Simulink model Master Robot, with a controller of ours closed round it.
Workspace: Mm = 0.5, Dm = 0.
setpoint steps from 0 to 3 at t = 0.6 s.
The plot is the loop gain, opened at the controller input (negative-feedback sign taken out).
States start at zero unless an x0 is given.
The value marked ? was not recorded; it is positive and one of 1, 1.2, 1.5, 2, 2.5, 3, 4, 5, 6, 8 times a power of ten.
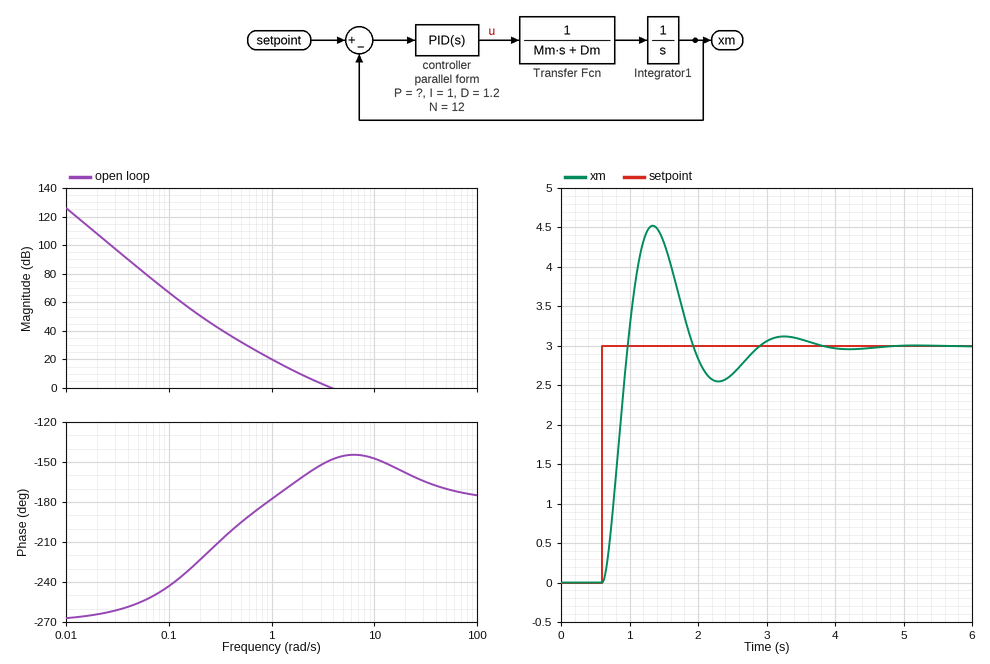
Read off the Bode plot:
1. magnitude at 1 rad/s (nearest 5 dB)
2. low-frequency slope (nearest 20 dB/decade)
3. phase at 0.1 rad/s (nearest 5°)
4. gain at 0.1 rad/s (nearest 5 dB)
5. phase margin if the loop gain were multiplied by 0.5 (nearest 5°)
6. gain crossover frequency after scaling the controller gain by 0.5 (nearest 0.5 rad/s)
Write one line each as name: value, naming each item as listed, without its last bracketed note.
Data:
magnitude at 1 rad/s: 20 dB
low-frequency slope: -60 dB/decade
phase at 0.1 rad/s: -245°
gain at 0.1 rad/s: 65 dB
phase margin if the loop gain were multiplied by 0.5: 25°
gain crossover frequency after scaling the controller gain by 0.5: 2.5 rad/s
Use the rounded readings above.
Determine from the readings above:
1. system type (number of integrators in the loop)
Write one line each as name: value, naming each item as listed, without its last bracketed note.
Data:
system type: 3
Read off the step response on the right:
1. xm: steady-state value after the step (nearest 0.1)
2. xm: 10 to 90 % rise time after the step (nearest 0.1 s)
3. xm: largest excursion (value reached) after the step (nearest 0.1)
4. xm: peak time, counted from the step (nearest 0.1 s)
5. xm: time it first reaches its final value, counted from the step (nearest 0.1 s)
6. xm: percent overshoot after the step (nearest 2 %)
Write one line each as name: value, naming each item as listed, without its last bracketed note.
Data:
xm: steady-state value after the step: 3.0
xm: 10 to 90 % rise time after the step: 0.3 s
xm: largest excursion (value reached) after the step: 4.5
xm: peak time, counted from the step: 0.7 s
xm: time it first reaches its final value, counted from the step: 0.4 s
xm: percent overshoot after the step: 50 %
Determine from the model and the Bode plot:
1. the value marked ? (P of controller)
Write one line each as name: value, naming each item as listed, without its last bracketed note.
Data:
the value marked ?: 5
